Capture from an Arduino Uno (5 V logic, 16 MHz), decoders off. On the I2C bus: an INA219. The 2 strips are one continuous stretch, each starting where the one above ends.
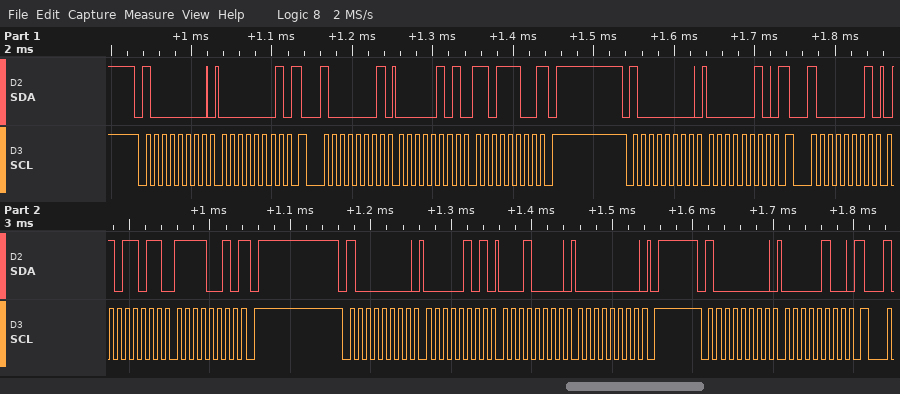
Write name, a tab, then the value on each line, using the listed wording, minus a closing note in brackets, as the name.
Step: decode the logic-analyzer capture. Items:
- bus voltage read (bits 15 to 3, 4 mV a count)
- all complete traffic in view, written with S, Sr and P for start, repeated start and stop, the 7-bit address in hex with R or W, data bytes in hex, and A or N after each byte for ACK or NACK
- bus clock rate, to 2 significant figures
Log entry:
bus voltage read	11.768 V
all complete traffic in view, written with S, Sr and P for start, repeated start and stop, the 7-bit address in hex with R or W, data bytes in hex, and A or N after each byte for ACK or NACK	S 40W A 01 A Sr 40R A 05 A DC N P S 40W A 02 A Sr 40R A 5B A F2 N P S 40W A 05 A 10 A 00 A P S 40W A 04 A
bus clock rate, to 2 significant figures	100 kHz
